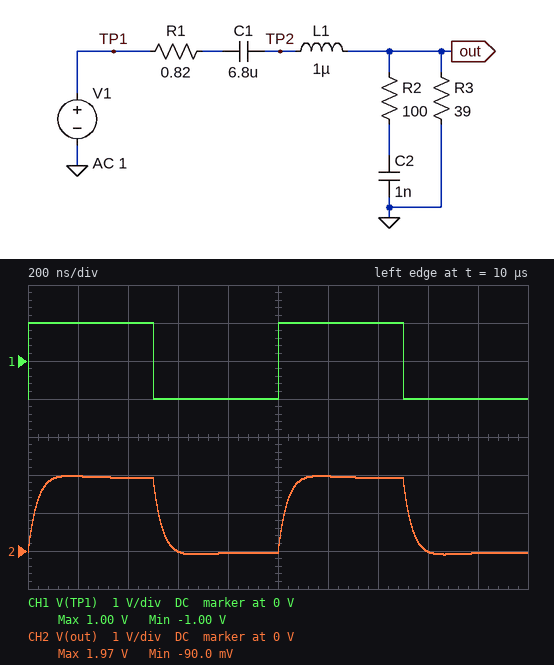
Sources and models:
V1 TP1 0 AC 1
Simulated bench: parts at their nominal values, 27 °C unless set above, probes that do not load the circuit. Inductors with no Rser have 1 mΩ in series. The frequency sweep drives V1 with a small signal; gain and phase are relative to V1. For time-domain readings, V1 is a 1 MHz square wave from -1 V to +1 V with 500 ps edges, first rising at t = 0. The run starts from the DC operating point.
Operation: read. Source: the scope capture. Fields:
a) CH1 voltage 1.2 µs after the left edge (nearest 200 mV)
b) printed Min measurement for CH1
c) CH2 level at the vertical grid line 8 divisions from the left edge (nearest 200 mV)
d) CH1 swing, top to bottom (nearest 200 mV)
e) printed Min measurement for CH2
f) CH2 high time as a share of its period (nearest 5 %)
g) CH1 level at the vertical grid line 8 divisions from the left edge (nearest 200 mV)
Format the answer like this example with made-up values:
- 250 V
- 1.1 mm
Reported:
- 1.0 V
- -1.00 V
- 0 V
- 2.0 V
- -90.0 mV
- 50 %
- -1.0 V
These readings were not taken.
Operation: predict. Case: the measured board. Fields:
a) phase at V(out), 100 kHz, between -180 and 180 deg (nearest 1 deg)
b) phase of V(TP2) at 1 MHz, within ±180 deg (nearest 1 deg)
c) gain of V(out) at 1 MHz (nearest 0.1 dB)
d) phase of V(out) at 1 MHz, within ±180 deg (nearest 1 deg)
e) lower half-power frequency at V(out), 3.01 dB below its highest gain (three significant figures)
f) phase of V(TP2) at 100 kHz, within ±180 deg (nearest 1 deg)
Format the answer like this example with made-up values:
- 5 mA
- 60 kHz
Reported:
- -1 deg
- 0 deg
- -0.1 dB
- -10 deg
- 599 Hz
- 0 deg
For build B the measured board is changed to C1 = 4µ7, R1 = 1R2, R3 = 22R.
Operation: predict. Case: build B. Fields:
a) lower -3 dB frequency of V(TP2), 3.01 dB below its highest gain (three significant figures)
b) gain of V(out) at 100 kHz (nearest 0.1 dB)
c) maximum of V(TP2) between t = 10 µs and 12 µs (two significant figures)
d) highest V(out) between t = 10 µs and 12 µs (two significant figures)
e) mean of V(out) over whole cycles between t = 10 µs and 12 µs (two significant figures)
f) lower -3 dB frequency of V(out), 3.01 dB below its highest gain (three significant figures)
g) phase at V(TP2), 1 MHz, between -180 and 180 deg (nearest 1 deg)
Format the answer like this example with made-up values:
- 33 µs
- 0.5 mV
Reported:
- 1.63 kHz
- -0.5 dB
- 1.9 V
- 1.8 V
- 860 mV
- 1.46 kHz
- 1 deg
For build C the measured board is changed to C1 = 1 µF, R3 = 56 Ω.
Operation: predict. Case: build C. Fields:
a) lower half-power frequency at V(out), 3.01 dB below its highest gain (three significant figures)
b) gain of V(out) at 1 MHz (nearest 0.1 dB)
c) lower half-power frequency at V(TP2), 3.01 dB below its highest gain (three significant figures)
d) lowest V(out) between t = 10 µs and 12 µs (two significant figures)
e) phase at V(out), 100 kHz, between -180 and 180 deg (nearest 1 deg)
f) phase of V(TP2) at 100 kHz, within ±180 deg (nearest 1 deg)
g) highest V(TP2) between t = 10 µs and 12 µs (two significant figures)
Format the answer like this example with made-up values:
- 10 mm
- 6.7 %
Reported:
- 2.92 kHz
- 0 dB
- 2.89 kHz
- -250 mV
- 1 deg
- 2 deg
- 1.8 V
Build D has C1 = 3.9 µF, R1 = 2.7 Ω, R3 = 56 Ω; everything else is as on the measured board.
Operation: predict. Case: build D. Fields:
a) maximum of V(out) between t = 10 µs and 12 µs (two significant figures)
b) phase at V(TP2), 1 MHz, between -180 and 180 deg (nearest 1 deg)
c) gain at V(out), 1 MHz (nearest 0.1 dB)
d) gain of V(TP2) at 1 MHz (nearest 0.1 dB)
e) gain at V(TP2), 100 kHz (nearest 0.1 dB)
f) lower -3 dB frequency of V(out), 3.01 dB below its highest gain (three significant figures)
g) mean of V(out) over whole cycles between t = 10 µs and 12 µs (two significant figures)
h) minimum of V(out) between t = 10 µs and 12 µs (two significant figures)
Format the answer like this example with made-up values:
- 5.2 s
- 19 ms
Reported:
- 1.9 V
- 0 deg
- -0.3 dB
- -0.5 dB
- -0.4 dB
- 711 Hz
- 910 mV
- -95 mV
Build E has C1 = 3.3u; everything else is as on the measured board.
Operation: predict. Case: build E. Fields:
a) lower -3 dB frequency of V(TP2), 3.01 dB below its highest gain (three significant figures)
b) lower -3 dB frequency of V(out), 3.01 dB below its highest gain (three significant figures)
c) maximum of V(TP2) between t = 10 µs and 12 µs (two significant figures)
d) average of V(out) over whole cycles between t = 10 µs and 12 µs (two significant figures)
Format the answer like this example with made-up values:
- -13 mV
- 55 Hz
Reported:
- 1.26 kHz
- 1.23 kHz
- 1.9 V
- 900 mV
